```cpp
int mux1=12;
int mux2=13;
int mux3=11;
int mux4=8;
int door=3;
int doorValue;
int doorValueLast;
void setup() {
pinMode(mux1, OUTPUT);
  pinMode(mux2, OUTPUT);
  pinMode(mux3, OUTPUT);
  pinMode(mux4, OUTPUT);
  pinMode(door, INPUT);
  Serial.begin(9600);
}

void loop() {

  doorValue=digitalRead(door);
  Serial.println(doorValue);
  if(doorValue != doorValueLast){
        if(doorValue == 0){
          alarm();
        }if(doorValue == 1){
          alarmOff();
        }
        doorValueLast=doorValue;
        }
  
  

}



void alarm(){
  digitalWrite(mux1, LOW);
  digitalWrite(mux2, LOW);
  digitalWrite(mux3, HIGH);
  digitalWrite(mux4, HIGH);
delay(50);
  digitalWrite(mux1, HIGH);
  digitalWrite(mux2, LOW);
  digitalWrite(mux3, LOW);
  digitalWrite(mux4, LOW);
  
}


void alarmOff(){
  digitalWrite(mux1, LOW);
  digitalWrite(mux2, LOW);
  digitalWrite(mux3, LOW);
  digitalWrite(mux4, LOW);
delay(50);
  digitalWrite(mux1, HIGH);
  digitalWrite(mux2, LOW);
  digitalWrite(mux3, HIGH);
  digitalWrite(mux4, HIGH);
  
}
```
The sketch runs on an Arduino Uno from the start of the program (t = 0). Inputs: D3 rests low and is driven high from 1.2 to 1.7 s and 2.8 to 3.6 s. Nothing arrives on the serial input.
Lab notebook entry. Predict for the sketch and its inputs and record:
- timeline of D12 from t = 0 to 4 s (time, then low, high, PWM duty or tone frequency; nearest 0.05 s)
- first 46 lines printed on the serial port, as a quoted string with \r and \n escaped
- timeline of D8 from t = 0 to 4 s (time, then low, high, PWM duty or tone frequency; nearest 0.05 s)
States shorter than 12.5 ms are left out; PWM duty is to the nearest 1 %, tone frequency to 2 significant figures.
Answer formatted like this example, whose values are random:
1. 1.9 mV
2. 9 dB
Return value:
1. 0 s low; 1.25 s high; 1.7 s low; 1.75 s high; 2.8 s low; 2.85 s high; 3.6 s low; 3.65 s high
2. "0\r\n0\r\n0\r\n0\r\n0\r\n0\r\n0\r\n0\r\n0\r\n0\r\n0\r\n0\r\n0\r\n0\r\n0\r\n0\r\n0\r\n0\r\n0\r\n0\r\n0\r\n0\r\n0\r\n0\r\n0\r\n0\r\n0\r\n0\r\n0\r\n0\r\n0\r\n0\r\n0\r\n0\r\n0\r\n0\r\n0\r\n0\r\n0\r\n0\r\n0\r\n0\r\n0\r\n0\r\n0\r\n0\r\n"
3. 0 s low; 1.25 s high; 1.75 s low; 2.85 s high; 3.65 s low
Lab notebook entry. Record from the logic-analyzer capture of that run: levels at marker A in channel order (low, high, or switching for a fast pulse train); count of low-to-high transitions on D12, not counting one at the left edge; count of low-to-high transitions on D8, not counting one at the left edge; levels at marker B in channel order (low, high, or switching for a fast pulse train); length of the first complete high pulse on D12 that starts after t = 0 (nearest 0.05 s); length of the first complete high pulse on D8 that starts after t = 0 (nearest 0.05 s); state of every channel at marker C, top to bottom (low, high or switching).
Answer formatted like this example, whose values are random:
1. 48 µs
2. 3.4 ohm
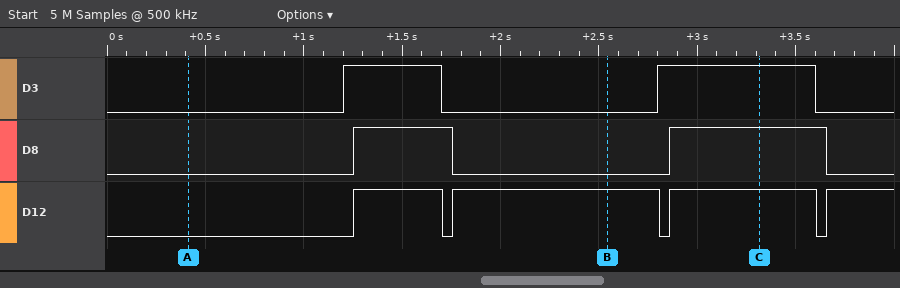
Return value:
1. D3 low, D8 low, D12 low
2. 4
3. 2
4. D3 low, D8 low, D12 high
5. 0.45 s
6. 0.50 s
7. D3 high, D8 high, D12 high
